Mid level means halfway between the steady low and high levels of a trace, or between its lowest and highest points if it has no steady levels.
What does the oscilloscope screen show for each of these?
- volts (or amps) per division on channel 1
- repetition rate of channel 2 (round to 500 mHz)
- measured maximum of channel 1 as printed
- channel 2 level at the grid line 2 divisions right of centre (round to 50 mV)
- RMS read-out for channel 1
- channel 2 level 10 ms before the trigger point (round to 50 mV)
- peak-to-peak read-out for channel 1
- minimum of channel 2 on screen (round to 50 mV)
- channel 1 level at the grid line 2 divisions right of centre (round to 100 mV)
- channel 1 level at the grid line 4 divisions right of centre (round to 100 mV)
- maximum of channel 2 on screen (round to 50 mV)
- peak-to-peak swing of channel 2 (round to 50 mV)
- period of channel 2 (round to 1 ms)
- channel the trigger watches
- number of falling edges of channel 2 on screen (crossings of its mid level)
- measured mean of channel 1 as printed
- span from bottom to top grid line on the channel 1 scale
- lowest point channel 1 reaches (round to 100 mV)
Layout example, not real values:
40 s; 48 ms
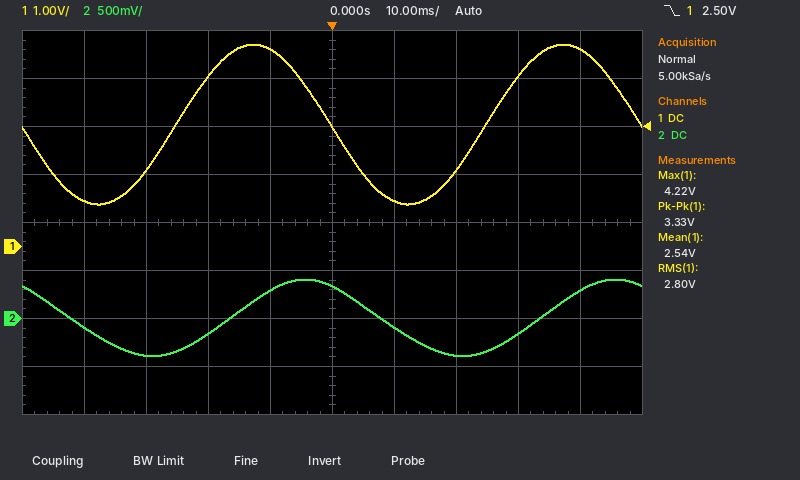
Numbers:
1 V; 20.0 Hz; 4.22 V; -400 mV; 2.80 V; 300 mV; 3.33 V; -400 mV; 1.6 V; 4.1 V; 400 mV; 800 mV; 50 ms; channel 1; 2; 2.54 V; 8 V; 900 mV
